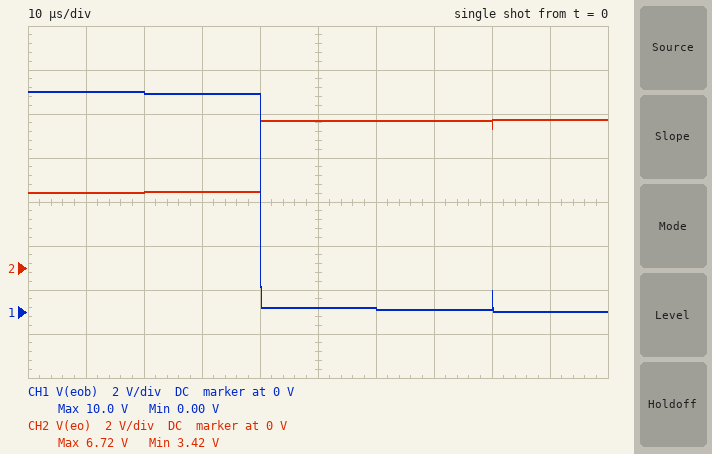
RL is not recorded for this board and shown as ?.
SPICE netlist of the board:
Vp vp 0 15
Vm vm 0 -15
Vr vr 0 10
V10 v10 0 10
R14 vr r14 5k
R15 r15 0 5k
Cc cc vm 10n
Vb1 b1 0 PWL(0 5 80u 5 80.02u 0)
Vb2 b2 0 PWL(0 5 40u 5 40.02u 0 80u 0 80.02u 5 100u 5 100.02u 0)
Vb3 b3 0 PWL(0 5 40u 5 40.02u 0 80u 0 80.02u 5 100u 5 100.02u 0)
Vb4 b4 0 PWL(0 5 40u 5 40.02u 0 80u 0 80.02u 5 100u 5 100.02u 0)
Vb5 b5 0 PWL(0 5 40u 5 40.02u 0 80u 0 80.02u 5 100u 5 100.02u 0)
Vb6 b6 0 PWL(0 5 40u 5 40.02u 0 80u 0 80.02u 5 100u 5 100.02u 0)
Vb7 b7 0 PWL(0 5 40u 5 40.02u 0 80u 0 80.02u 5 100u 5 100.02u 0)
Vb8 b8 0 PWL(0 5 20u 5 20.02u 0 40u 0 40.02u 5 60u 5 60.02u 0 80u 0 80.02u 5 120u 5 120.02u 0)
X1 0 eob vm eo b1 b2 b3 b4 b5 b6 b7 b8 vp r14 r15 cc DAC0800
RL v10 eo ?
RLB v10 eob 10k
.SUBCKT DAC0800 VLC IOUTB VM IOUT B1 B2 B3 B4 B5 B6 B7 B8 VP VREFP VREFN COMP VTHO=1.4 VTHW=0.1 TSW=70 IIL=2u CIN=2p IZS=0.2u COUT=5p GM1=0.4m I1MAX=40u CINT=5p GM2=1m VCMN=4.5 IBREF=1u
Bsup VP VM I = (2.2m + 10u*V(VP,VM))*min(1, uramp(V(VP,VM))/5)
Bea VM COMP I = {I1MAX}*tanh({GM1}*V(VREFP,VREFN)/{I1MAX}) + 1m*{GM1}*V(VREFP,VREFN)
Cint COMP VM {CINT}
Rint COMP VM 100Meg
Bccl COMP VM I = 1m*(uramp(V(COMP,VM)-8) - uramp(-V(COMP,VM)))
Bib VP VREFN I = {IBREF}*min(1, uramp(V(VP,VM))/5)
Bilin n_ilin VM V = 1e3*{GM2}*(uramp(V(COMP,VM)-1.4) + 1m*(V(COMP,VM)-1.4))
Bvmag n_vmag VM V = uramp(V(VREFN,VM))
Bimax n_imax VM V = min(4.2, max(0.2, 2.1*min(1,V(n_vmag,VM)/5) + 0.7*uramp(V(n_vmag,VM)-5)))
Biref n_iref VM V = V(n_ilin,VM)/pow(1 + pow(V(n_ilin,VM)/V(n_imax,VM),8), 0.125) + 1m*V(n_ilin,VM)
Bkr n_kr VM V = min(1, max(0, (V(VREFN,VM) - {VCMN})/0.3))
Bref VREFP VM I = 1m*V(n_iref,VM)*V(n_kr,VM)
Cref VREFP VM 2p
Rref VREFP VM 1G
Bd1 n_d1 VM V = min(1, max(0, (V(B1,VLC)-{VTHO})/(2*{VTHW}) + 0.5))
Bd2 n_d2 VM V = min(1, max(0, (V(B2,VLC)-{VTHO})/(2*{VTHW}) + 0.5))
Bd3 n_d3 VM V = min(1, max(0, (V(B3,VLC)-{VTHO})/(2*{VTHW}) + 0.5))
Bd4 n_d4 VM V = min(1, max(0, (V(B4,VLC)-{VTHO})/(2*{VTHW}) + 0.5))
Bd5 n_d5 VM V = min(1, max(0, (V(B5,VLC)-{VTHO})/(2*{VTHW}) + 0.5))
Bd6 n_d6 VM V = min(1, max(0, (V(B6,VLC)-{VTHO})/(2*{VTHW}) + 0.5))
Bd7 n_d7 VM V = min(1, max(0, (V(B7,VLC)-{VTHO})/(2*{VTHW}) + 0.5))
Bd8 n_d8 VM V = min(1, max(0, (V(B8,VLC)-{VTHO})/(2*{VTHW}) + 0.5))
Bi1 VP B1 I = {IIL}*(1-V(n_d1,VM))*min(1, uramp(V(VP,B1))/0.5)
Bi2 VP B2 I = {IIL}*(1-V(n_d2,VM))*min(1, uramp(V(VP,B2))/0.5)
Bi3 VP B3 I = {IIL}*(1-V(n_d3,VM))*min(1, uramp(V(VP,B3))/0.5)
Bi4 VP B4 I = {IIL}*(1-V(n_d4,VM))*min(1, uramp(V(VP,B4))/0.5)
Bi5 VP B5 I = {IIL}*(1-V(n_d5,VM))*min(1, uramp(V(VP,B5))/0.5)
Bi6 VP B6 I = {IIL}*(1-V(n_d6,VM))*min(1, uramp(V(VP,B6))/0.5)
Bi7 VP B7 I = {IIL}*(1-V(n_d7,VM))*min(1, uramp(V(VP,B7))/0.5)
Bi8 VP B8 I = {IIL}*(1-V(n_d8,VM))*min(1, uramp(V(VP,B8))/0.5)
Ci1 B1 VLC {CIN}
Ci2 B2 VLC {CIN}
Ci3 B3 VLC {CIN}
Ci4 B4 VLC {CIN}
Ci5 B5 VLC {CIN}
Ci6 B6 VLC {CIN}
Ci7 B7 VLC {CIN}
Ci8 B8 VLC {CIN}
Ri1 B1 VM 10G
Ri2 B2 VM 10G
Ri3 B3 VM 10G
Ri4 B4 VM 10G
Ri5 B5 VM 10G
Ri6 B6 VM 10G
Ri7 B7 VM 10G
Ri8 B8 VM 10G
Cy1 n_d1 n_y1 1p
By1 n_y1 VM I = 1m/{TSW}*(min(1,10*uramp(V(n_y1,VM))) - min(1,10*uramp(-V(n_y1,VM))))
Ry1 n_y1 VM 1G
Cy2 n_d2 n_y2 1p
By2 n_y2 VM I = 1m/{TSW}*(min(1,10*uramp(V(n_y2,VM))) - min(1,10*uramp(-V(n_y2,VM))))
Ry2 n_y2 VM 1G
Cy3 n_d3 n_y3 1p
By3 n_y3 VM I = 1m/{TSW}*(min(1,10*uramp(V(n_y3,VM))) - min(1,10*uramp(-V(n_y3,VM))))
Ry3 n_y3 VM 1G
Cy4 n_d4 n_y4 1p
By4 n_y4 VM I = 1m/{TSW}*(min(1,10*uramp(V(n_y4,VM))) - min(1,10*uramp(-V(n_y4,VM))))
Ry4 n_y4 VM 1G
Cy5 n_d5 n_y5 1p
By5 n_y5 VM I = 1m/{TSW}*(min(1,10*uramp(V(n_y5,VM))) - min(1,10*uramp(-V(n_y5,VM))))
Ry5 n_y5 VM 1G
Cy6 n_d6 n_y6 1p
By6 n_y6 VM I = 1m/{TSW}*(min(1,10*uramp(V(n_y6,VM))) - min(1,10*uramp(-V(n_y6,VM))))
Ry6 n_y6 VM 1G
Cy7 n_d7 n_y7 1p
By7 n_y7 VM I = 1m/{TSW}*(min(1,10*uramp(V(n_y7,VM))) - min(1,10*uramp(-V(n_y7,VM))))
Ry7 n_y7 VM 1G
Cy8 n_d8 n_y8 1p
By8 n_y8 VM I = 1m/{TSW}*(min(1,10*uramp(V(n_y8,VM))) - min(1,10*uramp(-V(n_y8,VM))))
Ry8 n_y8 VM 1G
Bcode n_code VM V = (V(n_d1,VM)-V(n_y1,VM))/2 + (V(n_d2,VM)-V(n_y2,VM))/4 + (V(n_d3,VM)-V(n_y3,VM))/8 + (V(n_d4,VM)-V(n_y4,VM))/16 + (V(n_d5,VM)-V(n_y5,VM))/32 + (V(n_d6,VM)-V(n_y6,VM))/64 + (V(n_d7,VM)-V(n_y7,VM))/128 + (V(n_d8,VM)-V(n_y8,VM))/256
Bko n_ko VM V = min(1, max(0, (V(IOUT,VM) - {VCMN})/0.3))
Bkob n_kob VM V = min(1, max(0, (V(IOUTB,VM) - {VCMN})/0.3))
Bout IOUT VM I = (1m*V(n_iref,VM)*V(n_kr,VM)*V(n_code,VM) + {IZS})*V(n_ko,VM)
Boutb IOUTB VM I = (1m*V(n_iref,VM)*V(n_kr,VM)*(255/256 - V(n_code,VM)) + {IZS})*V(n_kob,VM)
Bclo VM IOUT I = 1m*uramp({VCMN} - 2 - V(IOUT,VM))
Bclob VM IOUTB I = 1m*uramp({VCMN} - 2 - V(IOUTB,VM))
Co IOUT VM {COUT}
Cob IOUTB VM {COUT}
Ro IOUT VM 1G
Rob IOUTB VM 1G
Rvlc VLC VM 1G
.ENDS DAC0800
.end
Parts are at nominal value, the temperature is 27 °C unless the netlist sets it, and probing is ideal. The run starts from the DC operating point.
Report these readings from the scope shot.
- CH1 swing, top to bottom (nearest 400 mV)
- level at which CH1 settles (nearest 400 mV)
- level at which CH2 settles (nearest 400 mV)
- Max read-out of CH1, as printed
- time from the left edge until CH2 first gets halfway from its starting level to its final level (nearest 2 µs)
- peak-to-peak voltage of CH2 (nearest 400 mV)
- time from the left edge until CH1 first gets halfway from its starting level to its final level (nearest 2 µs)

10.0 V
0 V
6.8 V
10.0 V
40 µs
3.2 V
40 µs
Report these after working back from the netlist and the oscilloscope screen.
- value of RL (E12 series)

3.3 kΩ
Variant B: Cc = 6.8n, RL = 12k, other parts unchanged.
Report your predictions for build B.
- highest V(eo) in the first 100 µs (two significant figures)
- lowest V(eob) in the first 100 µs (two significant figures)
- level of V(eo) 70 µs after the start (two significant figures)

-1.9 V
3.0 mV
-2.0 V
